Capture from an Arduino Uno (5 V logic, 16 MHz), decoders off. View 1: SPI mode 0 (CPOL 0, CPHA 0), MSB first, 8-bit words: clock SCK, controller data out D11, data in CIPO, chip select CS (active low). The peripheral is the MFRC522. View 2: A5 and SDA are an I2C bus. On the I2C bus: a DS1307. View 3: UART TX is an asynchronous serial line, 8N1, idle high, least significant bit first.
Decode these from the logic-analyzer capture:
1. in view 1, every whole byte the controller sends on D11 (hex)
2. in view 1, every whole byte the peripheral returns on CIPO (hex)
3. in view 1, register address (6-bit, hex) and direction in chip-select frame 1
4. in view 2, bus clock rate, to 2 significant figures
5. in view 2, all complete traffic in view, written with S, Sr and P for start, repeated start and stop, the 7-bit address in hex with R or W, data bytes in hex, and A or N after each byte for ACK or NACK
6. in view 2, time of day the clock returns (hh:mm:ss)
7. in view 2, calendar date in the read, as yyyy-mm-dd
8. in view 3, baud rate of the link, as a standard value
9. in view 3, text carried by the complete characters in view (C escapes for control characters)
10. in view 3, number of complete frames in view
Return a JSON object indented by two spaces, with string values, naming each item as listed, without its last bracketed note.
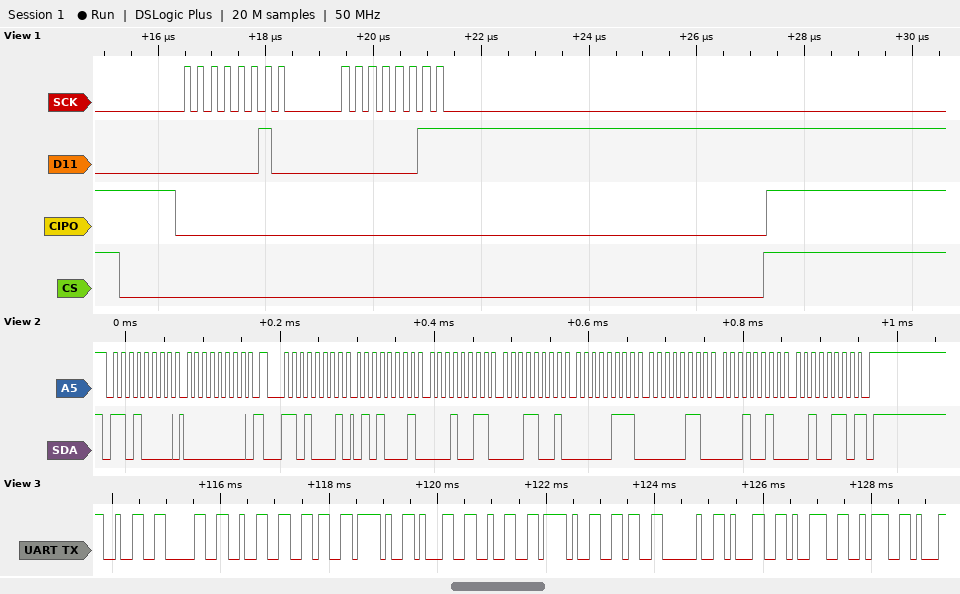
{
  "in view 1, every whole byte the controller sends on D11": "0x02 0x03",
  "in view 1, every whole byte the peripheral returns on CIPO": "0x00 0x00",
  "in view 1, register address (6-bit, hex) and direction in chip-select frame 1": "0x01 write",
  "in view 2, bus clock rate, to 2 significant figures": "100 kHz",
  "in view 2, all complete traffic in view, written with S, Sr and P for start, repeated start and stop, the 7-bit address in hex with R or W, data bytes in hex, and A or N after each byte for ACK or NACK": "S 68W A 00 A Sr 68R A 51 A 13 A 19 A 07 A 06 A 12 A 26 N P",
  "in view 2, time of day the clock returns": "19:13:51",
  "in view 2, calendar date in the read, as yyyy-mm-dd": "2026-12-06",
  "in view 3, baud rate of the link, as a standard value": "9600 baud",
  "in view 3, text carried by the complete characters in view": "\"2026/12/6 19:\"",
  "in view 3, number of complete frames in view": "13"
}
